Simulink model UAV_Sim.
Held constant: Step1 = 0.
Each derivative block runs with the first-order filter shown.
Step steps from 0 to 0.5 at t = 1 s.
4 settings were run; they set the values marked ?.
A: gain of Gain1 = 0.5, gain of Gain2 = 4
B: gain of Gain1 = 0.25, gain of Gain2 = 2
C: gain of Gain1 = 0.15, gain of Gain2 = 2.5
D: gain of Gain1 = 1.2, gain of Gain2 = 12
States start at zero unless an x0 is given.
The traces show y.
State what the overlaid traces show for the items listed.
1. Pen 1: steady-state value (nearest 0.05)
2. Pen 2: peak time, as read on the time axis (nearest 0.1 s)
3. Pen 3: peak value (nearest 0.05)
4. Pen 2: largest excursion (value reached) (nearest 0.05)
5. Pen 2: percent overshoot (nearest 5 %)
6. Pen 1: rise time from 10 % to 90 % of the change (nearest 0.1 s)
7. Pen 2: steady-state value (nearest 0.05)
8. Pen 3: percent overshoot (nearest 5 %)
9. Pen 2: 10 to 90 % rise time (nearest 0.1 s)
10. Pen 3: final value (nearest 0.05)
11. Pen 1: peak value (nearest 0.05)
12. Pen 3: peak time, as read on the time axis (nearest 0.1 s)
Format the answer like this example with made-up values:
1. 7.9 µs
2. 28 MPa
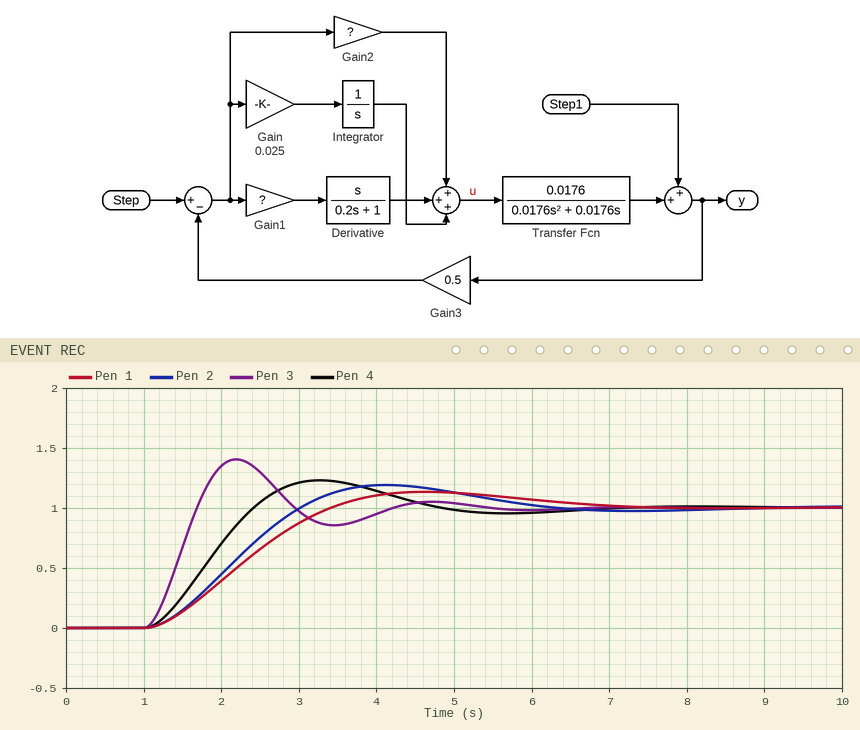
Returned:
1. 1.00
2. 4.1 s
3. 1.40
4. 1.20
5. 20 %
6. 1.7 s
7. 1.00
8. 40 %
9. 1.4 s
10. 1.00
11. 1.15
12. 2.2 s
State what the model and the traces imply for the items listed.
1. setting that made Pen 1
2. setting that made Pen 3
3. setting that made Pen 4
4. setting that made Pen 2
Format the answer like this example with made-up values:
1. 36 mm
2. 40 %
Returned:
1. B
2. D
3. A
4. C
